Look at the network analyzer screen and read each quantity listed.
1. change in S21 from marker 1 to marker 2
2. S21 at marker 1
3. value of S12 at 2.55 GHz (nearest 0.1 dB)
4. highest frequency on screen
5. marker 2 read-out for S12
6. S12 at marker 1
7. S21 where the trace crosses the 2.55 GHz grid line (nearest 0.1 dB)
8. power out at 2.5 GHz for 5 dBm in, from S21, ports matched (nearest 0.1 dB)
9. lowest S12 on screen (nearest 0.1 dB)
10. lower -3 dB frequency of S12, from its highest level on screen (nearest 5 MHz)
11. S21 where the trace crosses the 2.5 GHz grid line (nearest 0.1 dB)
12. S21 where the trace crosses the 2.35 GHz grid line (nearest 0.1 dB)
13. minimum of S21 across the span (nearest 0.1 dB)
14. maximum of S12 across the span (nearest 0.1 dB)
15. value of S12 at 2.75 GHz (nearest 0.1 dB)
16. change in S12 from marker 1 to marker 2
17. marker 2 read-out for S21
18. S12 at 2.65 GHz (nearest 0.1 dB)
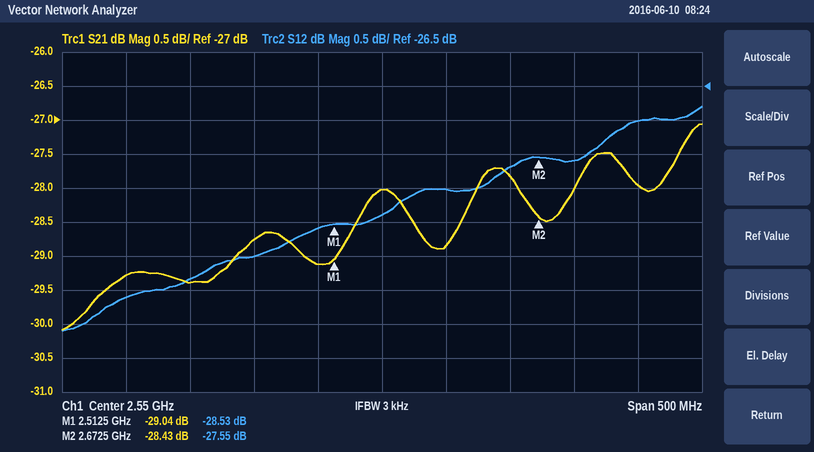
0.61 dB
-29.04 dB
-28.4 dB
2.8 GHz
-27.55 dB
-28.53 dB
-28.0 dB
-24.1 dBm
-30.1 dB
2.330 GHz
-29.1 dB
-29.3 dB
-30.1 dB
-26.8 dB
-27.0 dB
0.98 dB
-28.43 dB
-27.7 dB
